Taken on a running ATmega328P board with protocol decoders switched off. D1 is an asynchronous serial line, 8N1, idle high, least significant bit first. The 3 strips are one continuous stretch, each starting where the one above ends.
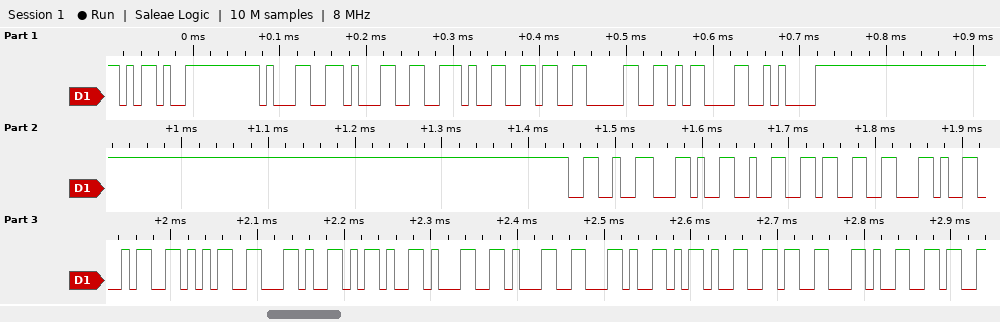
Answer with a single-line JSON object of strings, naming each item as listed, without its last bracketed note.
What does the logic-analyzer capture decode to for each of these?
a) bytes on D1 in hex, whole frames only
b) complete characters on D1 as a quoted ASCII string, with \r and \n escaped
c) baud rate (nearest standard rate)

{"bytes on D1 in hex, whole frames only": "2D 31 31 2E 36 30 0D 0A 26 2C 32 33 2C 34 35 2C 2D 31 31 2C 2D 36 2C 36", "complete characters on D1 as a quoted ASCII string, with \\r and \\n escaped": "\"-11.60\\r\\n&,23,45,-11,-6,6\"", "baud rate": "115200 baud"}
